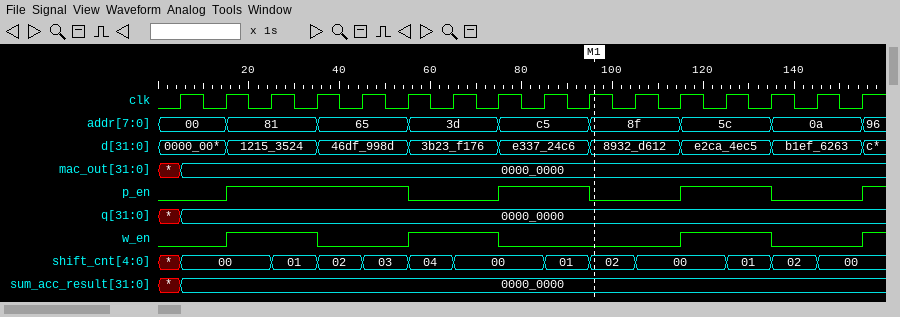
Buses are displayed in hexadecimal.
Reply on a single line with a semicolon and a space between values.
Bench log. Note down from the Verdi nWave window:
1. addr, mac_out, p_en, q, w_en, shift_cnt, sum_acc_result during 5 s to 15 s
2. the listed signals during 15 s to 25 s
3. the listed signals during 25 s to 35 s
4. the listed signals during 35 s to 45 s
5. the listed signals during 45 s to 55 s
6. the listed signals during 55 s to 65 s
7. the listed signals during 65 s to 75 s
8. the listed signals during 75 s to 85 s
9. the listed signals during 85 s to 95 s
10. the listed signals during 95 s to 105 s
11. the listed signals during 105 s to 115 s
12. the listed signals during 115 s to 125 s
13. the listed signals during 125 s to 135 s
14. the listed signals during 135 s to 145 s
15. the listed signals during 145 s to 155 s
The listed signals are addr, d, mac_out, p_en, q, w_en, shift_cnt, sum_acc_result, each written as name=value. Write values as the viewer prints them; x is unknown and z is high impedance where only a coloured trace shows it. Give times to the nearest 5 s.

addr=00, mac_out=0000_0000, p_en=0, q=0000_0000, w_en=0, shift_cnt=00, sum_acc_result=0000_0000; addr=81, d=1215_3524, mac_out=0000_0000, p_en=1, q=0000_0000, w_en=1, shift_cnt=00, sum_acc_result=0000_0000; addr=81, d=1215_3524, mac_out=0000_0000, p_en=1, q=0000_0000, w_en=1, shift_cnt=01, sum_acc_result=0000_0000; addr=65, d=46df_998d, mac_out=0000_0000, p_en=1, q=0000_0000, w_en=0, shift_cnt=02, sum_acc_result=0000_0000; addr=65, d=46df_998d, mac_out=0000_0000, p_en=1, q=0000_0000, w_en=0, shift_cnt=03, sum_acc_result=0000_0000; addr=3d, d=3b23_f176, mac_out=0000_0000, p_en=0, q=0000_0000, w_en=1, shift_cnt=04, sum_acc_result=0000_0000; addr=3d, d=3b23_f176, mac_out=0000_0000, p_en=0, q=0000_0000, w_en=1, shift_cnt=00, sum_acc_result=0000_0000; addr=c5, d=e337_24c6, mac_out=0000_0000, p_en=1, q=0000_0000, w_en=0, shift_cnt=00, sum_acc_result=0000_0000; addr=c5, d=e337_24c6, mac_out=0000_0000, p_en=1, q=0000_0000, w_en=0, shift_cnt=01, sum_acc_result=0000_0000; addr=8f, d=8932_d612, mac_out=0000_0000, p_en=0, q=0000_0000, w_en=0, shift_cnt=02, sum_acc_result=0000_0000; addr=8f, d=8932_d612, mac_out=0000_0000, p_en=0, q=0000_0000, w_en=0, shift_cnt=00, sum_acc_result=0000_0000; addr=5c, d=e2ca_4ec5, mac_out=0000_0000, p_en=1, q=0000_0000, w_en=1, shift_cnt=00, sum_acc_result=0000_0000; addr=5c, d=e2ca_4ec5, mac_out=0000_0000, p_en=1, q=0000_0000, w_en=1, shift_cnt=01, sum_acc_result=0000_0000; addr=0a, d=b1ef_6263, mac_out=0000_0000, p_en=0, q=0000_0000, w_en=0, shift_cnt=02, sum_acc_result=0000_0000; addr=0a, d=b1ef_6263, mac_out=0000_0000, p_en=0, q=0000_0000, w_en=0, shift_cnt=00, sum_acc_result=0000_0000
